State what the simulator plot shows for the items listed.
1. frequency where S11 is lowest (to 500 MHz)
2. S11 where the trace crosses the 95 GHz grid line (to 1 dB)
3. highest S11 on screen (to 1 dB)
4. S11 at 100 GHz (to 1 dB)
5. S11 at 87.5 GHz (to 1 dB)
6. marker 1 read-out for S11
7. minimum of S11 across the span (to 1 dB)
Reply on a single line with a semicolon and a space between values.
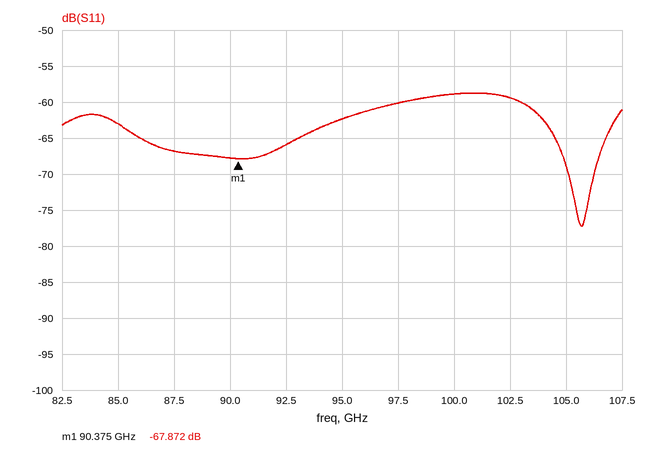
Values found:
105.5 GHz; -62 dB; -59 dB; -59 dB; -67 dB; -67.872 dB; -77 dB
